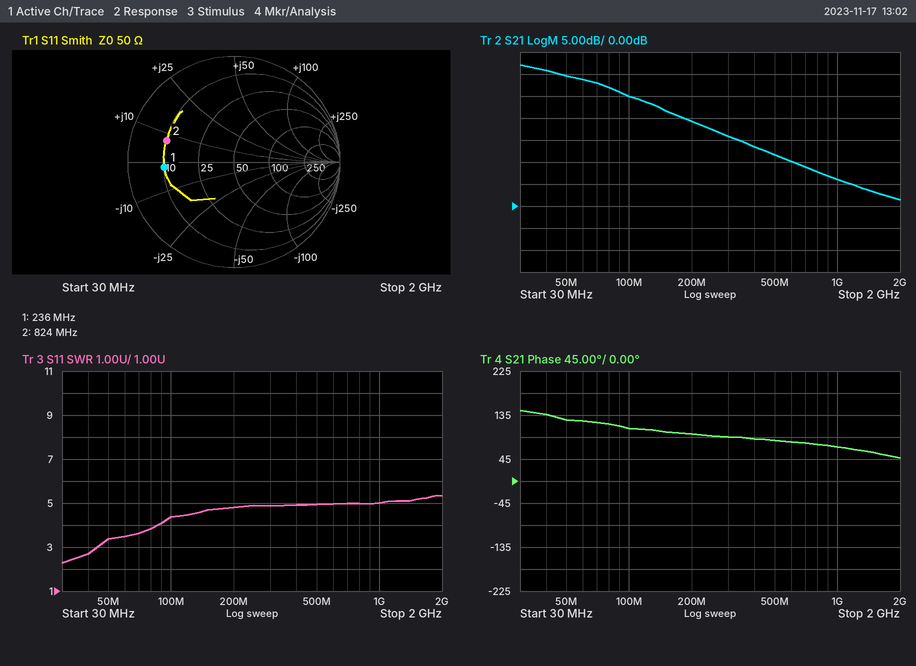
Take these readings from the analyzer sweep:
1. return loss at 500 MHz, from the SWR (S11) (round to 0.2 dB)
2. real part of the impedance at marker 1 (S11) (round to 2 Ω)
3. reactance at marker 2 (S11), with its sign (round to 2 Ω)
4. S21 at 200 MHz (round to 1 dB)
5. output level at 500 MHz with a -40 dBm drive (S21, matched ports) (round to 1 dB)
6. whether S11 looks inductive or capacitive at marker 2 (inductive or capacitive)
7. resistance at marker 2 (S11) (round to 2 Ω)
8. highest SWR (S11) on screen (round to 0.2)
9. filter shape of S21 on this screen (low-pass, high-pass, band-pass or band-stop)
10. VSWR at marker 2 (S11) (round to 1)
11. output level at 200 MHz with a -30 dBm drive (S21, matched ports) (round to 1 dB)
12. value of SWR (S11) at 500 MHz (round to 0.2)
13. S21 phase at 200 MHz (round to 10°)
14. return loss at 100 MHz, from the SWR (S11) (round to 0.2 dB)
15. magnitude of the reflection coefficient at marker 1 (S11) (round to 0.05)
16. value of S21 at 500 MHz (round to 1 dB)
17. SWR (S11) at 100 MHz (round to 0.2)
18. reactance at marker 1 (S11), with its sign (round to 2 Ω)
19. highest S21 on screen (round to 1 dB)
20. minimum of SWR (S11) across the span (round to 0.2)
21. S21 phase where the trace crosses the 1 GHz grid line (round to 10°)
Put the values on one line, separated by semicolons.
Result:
3.6 dB; 10 Ω; +8 Ω; 19 dB; -28 dBm; inductive; 10 Ω; 5.4; low-pass; 5; -11 dBm; 5.0; 100°; 4.0 dB; 0.65; 12 dB; 4.4; -2 Ω; 32 dB; 2.2; 70°
